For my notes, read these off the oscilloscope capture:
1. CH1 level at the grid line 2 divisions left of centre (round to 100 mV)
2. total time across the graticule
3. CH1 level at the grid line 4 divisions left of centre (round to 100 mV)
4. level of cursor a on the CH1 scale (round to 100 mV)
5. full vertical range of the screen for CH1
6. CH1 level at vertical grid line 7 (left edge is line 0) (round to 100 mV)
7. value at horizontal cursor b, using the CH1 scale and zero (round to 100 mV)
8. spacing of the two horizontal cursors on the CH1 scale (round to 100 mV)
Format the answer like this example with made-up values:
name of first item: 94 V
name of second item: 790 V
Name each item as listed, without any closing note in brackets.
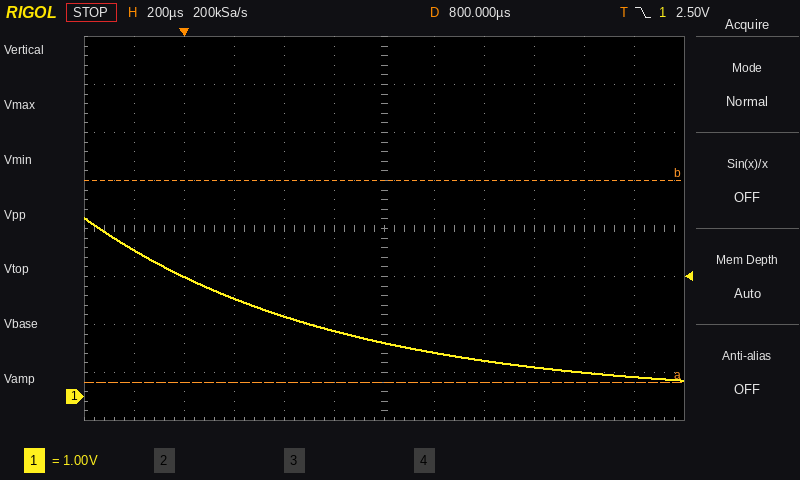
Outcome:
CH1 level at the grid line 2 divisions left of centre: 1.7 V
total time across the graticule: 2.4 ms
CH1 level at the grid line 4 divisions left of centre: 2.5 V
level of cursor a on the CH1 scale: 300 mV
full vertical range of the screen for CH1: 8 V
CH1 level at vertical grid line 7 (left edge is line 0): 900 mV
value at horizontal cursor b, using the CH1 scale and zero: 4.5 V
spacing of the two horizontal cursors on the CH1 scale: 4.2 V
